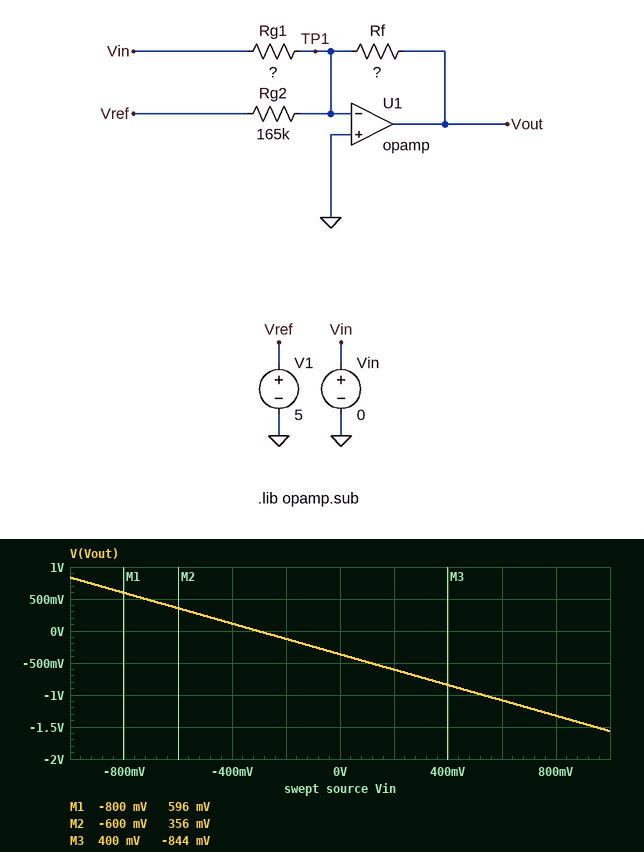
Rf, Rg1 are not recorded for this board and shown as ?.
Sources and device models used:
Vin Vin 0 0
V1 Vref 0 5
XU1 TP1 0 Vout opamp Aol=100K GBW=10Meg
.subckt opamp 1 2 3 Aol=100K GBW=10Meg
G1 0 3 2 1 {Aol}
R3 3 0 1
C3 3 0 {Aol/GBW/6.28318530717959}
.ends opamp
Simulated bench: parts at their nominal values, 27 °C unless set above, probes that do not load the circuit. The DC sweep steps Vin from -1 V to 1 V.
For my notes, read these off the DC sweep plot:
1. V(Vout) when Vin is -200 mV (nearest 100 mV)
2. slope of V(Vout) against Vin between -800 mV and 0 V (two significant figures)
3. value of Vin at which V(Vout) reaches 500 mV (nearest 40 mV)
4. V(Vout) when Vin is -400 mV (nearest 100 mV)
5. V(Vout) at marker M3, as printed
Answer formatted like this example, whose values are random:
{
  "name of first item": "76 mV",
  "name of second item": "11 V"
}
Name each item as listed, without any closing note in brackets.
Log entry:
{
  "V(Vout) when Vin is -200 mV": "-100 mV",
  "slope of V(Vout) against Vin between -800 mV and 0 V": "-1.2 V/V",
  "value of Vin at which V(Vout) reaches 500 mV": "-720 mV",
  "V(Vout) when Vin is -400 mV": "100 mV",
  "V(Vout) at marker M3, as printed": "-844 mV"
}
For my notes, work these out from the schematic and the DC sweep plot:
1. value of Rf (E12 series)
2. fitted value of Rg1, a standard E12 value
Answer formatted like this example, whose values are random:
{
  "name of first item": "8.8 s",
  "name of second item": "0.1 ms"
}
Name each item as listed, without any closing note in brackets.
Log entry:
{
  "value of Rf": "12 kΩ",
  "fitted value of Rg1, a standard E12 value": "10 kΩ"
}
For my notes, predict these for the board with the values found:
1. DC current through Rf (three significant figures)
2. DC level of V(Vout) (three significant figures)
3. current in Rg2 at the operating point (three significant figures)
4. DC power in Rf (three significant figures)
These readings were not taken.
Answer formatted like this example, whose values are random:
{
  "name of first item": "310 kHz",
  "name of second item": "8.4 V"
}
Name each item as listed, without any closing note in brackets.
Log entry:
{
  "DC current through Rf": "30.3 µA",
  "DC level of V(Vout)": "-364 mV",
  "current in Rg2 at the operating point": "30.3 µA",
  "DC power in Rf": "11.0 µW"
}
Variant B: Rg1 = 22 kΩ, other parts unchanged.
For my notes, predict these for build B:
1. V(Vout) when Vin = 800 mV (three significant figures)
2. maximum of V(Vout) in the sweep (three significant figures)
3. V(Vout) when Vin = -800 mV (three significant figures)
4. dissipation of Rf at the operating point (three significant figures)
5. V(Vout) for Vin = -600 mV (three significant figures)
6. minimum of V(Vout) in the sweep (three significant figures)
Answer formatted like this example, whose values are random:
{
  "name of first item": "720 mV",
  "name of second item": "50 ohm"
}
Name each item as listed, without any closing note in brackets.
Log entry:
{
  "V(Vout) when Vin = 800 mV": "-800 mV",
  "maximum of V(Vout) in the sweep": "182 mV",
  "V(Vout) when Vin = -800 mV": "72.7 mV",
  "dissipation of Rf at the operating point": "11.0 µW",
  "V(Vout) for Vin = -600 mV": "-36.4 mV",
  "minimum of V(Vout) in the sweep": "-909 mV"
}
